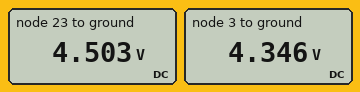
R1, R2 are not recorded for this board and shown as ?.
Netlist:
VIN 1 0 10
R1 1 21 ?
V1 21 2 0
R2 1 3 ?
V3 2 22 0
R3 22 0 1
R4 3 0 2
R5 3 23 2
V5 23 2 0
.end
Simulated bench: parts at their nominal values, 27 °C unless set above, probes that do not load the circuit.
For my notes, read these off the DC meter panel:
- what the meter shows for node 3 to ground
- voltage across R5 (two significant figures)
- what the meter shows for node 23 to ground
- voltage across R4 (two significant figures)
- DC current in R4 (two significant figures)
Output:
4.346 V
160 mV
4.503 V
4.3 V
2.2 A
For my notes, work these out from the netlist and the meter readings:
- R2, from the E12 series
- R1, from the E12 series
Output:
2.7 Ω
1.2 Ω
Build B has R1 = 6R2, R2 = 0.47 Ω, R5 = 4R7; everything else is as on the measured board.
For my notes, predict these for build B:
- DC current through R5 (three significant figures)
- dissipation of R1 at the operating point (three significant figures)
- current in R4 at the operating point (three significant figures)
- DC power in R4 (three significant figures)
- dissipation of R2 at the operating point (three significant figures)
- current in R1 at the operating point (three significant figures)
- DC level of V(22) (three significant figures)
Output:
1.13 A
9.41 W
3.83 A
29.4 W
11.6 W
1.23 A
2.36 V
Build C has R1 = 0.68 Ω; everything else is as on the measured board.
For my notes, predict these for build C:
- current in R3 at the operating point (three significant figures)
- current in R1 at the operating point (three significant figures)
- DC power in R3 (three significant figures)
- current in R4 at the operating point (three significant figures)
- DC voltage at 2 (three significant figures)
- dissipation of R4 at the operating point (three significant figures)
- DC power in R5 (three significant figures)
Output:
5.76 A
6.24 A
33.2 W
2.40 A
5.76 V
11.5 W
456 mW
